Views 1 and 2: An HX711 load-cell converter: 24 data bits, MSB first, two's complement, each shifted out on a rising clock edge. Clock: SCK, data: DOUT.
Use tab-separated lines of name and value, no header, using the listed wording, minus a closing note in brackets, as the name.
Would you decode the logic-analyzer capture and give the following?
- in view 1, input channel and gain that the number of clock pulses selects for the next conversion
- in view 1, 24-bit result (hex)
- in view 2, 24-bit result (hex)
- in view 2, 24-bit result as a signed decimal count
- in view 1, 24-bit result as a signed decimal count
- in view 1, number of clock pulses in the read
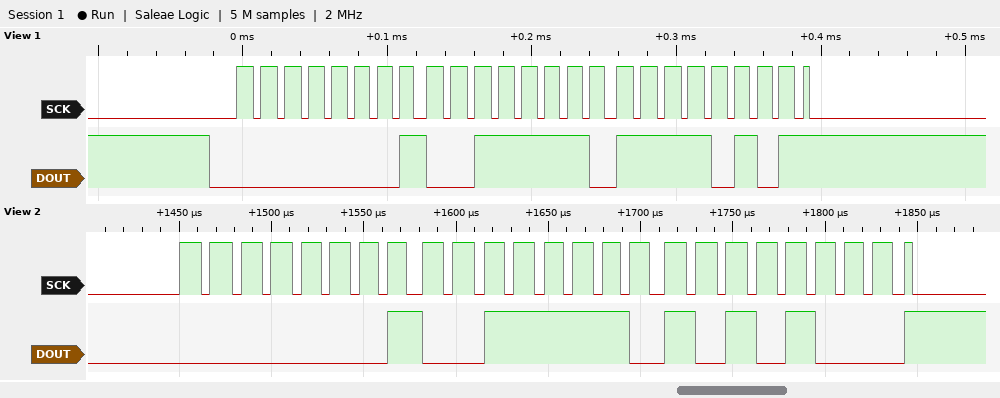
in view 1, input channel and gain that the number of clock pulses selects for the next conversion	channel A, gain 128
in view 1, 24-bit result	0x013EF5
in view 2, 24-bit result	0x013EA8
in view 2, 24-bit result as a signed decimal count	81576
in view 1, 24-bit result as a signed decimal count	81653
in view 1, number of clock pulses in the read	25
